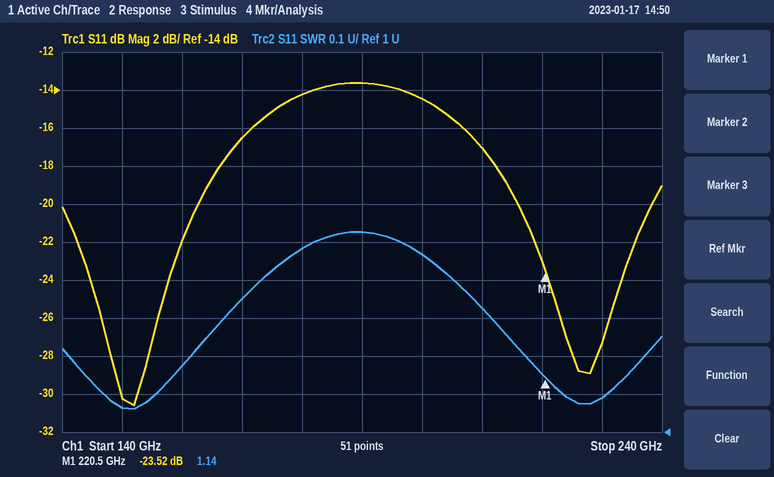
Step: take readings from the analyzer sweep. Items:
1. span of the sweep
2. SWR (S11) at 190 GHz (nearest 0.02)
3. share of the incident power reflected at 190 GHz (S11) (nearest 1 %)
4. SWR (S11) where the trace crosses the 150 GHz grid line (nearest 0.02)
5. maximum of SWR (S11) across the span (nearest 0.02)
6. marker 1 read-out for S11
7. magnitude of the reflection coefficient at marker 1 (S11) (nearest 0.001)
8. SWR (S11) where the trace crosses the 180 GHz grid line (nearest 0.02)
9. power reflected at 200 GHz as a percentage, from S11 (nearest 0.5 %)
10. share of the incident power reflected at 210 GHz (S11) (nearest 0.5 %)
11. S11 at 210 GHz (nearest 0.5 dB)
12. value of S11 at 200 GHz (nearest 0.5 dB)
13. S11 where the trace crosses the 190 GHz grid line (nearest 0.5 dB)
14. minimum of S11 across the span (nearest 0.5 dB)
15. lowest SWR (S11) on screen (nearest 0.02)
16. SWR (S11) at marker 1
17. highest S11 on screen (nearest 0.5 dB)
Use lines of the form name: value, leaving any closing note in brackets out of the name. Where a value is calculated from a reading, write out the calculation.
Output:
span of the sweep: 100 GHz
SWR (S11) at 190 GHz: 1.52
share of the incident power reflected at 190 GHz (S11): 10^(-13.5/10) ≈ 4 %
SWR (S11) where the trace crosses the 150 GHz grid line: 1.06
maximum of SWR (S11) across the span: 1.52
marker 1 read-out for S11: -23.52 dB
magnitude of the reflection coefficient at marker 1 (S11): 10^(-23.52/20) ≈ 0.067
SWR (S11) where the trace crosses the 180 GHz grid line: 1.48
power reflected at 200 GHz as a percentage, from S11: 10^(-14.5/10) ≈ 3.5 %
share of the incident power reflected at 210 GHz (S11): 10^(-17/10) ≈ 2.0 %
S11 at 210 GHz: -17.0 dB
value of S11 at 200 GHz: -14.5 dB
S11 where the trace crosses the 190 GHz grid line: -13.5 dB
minimum of S11 across the span: -30.5 dB
lowest SWR (S11) on screen: 1.06
SWR (S11) at marker 1: 1.14
highest S11 on screen: -13.5 dB
